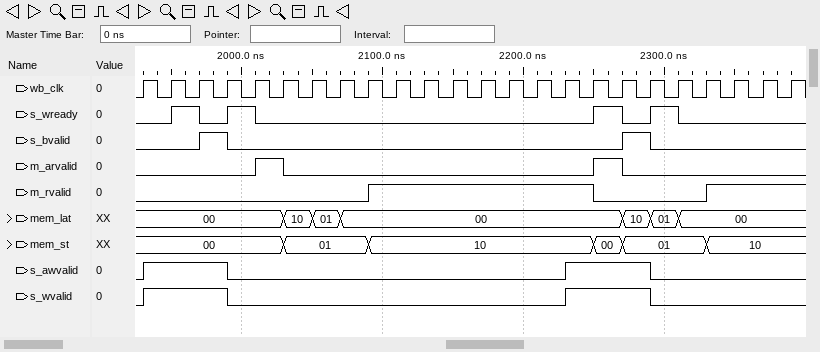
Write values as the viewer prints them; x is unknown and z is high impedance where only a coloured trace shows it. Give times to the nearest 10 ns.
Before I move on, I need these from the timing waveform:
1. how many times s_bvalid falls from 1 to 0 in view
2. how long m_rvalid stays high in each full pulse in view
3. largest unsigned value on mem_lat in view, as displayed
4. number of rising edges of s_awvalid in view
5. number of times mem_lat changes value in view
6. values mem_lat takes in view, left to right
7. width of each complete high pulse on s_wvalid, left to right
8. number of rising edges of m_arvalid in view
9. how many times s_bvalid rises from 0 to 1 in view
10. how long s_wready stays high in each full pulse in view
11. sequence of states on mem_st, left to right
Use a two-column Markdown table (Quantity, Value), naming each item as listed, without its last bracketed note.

| Quantity | Value |
|---|---|
| how many times s_bvalid falls from 1 to 0 in view | 2 |
| how long m_rvalid stays high in each full pulse in view | 160 ns |
| largest unsigned value on mem_lat in view, as displayed | 10 |
| number of rising edges of s_awvalid in view | 2 |
| number of times mem_lat changes value in view | 6 |
| values mem_lat takes in view, left to right | 00, 10, 01, 00, 10, 01, 00 |
| width of each complete high pulse on s_wvalid, left to right | 60 ns, 60 ns |
| number of rising edges of m_arvalid in view | 2 |
| how many times s_bvalid rises from 0 to 1 in view | 2 |
| how long s_wready stays high in each full pulse in view | 20 ns, 20 ns, 20 ns, 20 ns |
| sequence of states on mem_st, left to right | 00, 01, 10, 00, 01, 10 |
